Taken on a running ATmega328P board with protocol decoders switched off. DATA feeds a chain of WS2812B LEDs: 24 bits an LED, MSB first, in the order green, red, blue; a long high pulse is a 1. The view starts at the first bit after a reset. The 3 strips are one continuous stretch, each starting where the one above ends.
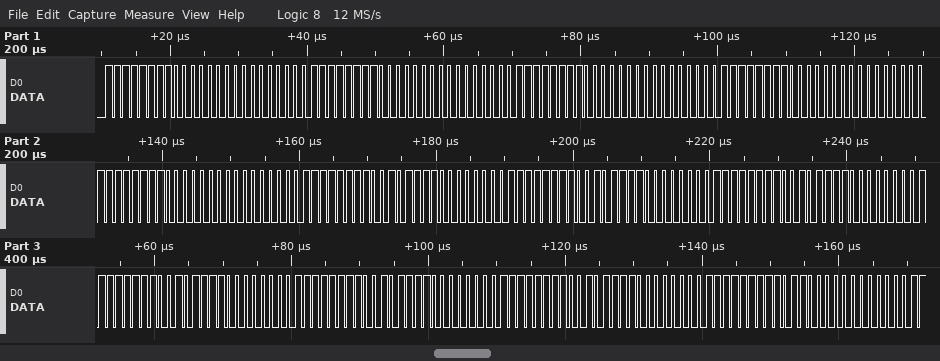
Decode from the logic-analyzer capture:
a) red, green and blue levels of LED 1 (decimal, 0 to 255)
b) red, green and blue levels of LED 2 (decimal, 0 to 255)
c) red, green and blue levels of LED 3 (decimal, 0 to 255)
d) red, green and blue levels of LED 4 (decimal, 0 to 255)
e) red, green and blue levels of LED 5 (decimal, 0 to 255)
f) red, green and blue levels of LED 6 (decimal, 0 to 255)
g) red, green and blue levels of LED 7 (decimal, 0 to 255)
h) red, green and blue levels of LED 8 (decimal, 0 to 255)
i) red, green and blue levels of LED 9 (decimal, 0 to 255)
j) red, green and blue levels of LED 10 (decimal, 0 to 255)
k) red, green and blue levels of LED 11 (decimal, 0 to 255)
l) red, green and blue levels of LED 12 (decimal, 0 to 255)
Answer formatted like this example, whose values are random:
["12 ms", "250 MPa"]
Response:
["0, 255, 0", "0, 255, 0", "0, 255, 0", "0, 255, 0", "0, 255, 0", "47, 255, 0", "47, 255, 0", "47, 255, 0", "47, 255, 0", "47, 255, 0", "47, 255, 0", "176, 255, 0"]
